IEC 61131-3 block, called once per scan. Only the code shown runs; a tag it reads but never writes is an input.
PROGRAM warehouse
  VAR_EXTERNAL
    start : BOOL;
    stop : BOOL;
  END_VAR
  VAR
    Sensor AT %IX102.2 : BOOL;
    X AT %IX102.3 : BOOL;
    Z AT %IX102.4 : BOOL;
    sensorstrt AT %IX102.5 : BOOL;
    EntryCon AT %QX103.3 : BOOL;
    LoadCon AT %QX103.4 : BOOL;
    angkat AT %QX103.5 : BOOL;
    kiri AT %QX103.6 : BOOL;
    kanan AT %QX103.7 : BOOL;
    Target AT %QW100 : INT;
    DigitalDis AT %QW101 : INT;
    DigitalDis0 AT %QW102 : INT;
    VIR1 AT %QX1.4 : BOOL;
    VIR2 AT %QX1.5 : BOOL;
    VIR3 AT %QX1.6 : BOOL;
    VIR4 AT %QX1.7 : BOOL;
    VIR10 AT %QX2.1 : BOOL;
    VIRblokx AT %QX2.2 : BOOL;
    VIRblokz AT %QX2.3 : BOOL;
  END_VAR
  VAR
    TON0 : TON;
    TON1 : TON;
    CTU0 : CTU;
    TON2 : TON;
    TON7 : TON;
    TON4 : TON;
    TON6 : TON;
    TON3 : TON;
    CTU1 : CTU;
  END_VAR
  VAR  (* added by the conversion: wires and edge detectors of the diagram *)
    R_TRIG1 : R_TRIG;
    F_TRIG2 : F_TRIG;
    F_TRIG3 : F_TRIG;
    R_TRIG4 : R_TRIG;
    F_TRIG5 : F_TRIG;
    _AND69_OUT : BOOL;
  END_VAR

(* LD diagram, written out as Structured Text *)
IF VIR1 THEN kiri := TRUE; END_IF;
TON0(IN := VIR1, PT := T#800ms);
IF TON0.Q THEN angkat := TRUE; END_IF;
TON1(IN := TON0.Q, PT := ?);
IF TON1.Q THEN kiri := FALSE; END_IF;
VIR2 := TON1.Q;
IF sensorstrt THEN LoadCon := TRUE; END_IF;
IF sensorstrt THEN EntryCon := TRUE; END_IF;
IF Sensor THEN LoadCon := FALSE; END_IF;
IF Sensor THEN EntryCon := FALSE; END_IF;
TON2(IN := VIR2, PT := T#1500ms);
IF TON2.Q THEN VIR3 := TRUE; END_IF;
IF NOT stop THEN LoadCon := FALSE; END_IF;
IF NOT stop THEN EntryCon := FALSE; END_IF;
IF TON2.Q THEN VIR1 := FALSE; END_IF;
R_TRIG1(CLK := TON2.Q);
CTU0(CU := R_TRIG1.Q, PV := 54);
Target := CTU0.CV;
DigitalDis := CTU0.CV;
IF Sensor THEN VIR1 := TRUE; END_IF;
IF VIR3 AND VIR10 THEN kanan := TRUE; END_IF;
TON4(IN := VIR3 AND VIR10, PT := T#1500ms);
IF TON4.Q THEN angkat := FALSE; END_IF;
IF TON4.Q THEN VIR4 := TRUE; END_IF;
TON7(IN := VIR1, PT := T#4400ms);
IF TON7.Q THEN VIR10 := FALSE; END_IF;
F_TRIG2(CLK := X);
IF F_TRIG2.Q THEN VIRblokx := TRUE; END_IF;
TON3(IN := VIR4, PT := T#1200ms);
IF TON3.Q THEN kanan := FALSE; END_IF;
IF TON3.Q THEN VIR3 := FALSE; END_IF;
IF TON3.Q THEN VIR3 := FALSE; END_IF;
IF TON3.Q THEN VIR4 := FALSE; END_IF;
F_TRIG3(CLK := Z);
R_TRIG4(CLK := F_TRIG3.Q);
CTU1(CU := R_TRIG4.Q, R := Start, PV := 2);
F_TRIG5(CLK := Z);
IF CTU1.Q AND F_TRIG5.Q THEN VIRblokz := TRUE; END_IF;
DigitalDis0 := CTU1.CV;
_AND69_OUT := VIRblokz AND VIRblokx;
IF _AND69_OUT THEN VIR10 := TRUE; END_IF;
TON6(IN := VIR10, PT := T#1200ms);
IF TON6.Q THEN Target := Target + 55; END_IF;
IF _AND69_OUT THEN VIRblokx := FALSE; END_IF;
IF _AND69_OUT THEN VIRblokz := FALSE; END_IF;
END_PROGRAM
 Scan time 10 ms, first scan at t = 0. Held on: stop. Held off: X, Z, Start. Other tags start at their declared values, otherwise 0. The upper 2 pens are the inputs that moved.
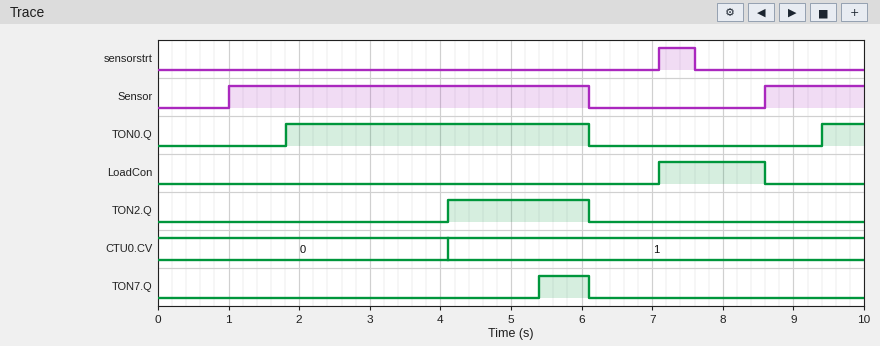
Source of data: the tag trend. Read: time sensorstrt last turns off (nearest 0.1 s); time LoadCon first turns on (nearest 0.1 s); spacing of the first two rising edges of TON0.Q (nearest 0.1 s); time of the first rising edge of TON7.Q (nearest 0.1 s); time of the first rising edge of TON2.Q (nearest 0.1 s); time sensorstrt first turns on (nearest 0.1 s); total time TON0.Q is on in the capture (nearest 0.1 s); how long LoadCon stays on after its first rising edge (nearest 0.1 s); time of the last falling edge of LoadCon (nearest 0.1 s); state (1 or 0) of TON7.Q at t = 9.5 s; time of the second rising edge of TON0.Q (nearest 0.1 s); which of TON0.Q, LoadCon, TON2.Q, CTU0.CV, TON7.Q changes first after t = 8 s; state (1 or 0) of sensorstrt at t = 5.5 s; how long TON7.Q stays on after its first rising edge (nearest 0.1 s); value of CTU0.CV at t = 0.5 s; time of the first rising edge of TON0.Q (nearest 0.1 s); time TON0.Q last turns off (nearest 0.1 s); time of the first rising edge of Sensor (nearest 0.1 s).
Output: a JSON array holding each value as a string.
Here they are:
["7.6 s", "7.1 s", "7.6 s", "5.4 s", "4.1 s", "7.1 s", "4.9 s", "1.5 s", "8.6 s", "0", "9.4 s", "LoadCon", "0", "0.7 s", "0", "1.8 s", "6.1 s", "1.0 s"]
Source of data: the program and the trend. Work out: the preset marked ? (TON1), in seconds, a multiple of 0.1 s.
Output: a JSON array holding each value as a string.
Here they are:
["0.8 s"]
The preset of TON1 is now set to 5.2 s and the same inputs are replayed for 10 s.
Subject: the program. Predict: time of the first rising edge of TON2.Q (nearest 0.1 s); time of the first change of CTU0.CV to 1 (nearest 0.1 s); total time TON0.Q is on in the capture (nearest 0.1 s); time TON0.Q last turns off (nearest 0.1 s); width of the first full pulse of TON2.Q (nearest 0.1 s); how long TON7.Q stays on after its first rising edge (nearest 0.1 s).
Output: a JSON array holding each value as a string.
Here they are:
["8.5 s", "8.5 s", "7.3 s", "8.5 s", "0.0 s", "3.1 s"]
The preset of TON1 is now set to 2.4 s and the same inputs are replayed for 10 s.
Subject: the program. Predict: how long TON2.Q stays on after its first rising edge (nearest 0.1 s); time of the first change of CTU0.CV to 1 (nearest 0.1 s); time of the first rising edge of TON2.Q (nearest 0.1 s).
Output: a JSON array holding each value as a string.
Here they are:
["0.4 s", "5.7 s", "5.7 s"]
